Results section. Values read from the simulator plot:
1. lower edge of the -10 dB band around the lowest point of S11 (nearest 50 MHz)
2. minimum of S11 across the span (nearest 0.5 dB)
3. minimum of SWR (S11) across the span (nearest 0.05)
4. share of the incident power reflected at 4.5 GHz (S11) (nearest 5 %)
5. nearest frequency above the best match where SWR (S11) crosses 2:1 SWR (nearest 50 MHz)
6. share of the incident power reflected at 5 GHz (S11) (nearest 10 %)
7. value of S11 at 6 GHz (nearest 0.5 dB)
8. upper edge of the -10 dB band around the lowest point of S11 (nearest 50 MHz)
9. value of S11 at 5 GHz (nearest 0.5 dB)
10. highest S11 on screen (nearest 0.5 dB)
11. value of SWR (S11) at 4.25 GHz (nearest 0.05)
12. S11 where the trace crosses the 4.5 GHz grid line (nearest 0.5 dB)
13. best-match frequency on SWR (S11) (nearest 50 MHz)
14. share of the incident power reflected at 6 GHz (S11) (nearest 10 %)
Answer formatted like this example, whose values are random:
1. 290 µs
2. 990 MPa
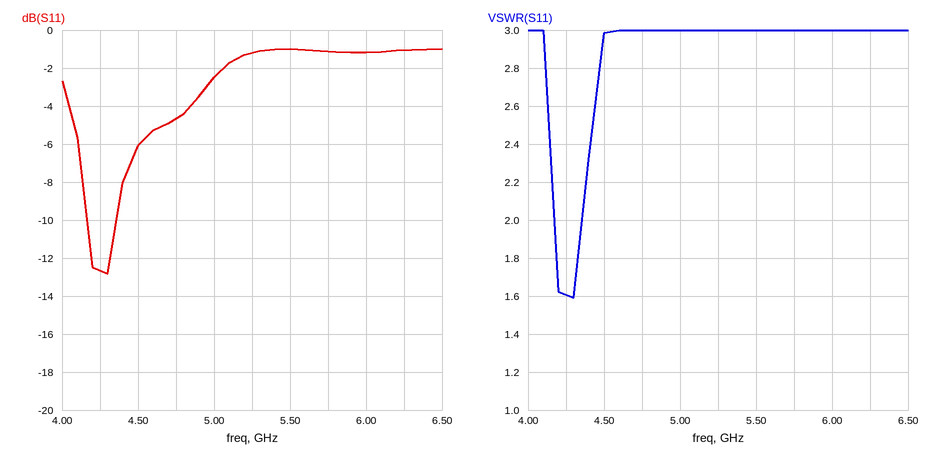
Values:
1. 4.15 GHz
2. -13.0 dB
3. 1.60
4. 25 %
5. 4.35 GHz
6. 60 %
7. -1.0 dB
8. 4.35 GHz
9. -2.5 dB
10. -1.0 dB
11. 1.60
12. -6.0 dB
13. 4.30 GHz
14. 80 %
